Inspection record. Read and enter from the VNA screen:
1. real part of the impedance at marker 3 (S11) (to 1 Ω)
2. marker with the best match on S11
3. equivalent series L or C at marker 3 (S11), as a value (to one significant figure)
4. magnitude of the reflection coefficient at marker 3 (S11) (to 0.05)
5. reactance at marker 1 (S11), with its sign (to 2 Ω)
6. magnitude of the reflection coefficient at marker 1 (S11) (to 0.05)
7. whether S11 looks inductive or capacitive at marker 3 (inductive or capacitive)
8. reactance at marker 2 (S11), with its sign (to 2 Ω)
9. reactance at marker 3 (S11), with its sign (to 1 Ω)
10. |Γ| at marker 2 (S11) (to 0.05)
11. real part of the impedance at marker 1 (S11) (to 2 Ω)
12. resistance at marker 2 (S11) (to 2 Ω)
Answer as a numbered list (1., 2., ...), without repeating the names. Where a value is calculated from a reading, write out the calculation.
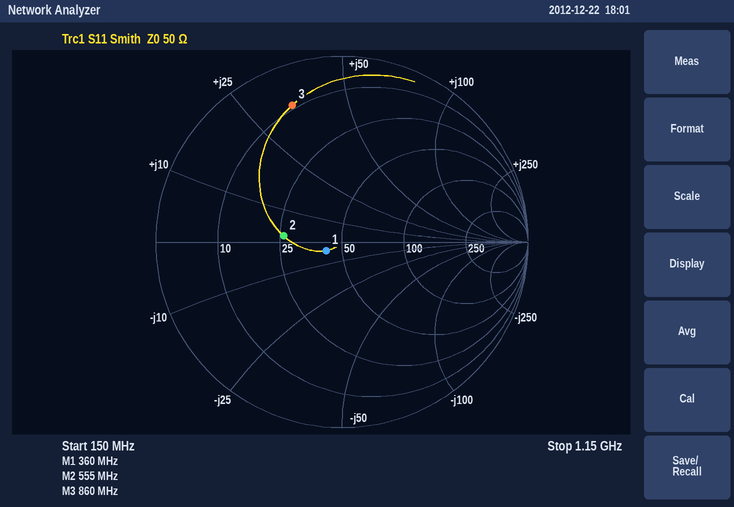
1. 9 Ω
2. marker 1
3. L = 34 Ω/(2π × 860 MHz) ≈ 6 nH
4. 0.80
5. -4 Ω
6. 0.10
7. inductive
8. +2 Ω
9. +34 Ω
10. 0.30
11. 42 Ω
12. 26 Ω
